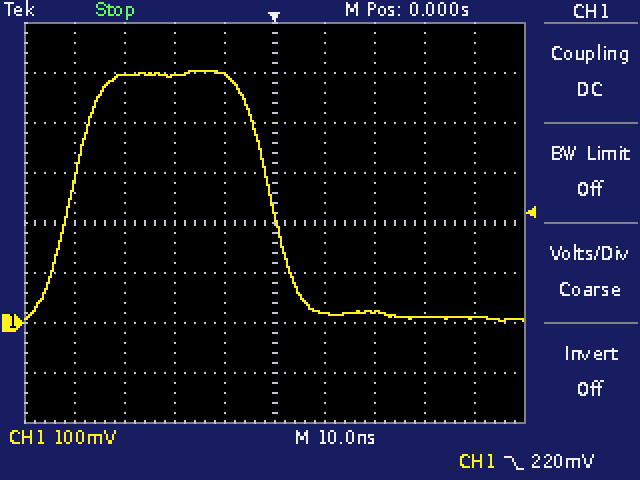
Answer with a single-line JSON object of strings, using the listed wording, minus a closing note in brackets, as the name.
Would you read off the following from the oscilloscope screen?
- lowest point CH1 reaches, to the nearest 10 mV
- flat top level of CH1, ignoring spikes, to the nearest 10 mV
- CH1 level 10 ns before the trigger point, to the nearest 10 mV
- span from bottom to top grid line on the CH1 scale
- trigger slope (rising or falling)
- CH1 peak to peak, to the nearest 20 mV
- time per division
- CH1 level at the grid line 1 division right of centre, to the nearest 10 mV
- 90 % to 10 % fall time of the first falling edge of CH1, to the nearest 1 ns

{"lowest point CH1 reaches, to the nearest 10 mV": "0 mV", "flat top level of CH1, ignoring spikes, to the nearest 10 mV": "500 mV", "CH1 level 10 ns before the trigger point, to the nearest 10 mV": "500 mV", "span from bottom to top grid line on the CH1 scale": "800 mV", "trigger slope": "falling", "CH1 peak to peak, to the nearest 20 mV": "500 mV", "time per division": "10 ns", "CH1 level at the grid line 1 division right of centre, to the nearest 10 mV": "20 mV", "90 % to 10 % fall time of the first falling edge of CH1, to the nearest 1 ns": "11 ns"}
